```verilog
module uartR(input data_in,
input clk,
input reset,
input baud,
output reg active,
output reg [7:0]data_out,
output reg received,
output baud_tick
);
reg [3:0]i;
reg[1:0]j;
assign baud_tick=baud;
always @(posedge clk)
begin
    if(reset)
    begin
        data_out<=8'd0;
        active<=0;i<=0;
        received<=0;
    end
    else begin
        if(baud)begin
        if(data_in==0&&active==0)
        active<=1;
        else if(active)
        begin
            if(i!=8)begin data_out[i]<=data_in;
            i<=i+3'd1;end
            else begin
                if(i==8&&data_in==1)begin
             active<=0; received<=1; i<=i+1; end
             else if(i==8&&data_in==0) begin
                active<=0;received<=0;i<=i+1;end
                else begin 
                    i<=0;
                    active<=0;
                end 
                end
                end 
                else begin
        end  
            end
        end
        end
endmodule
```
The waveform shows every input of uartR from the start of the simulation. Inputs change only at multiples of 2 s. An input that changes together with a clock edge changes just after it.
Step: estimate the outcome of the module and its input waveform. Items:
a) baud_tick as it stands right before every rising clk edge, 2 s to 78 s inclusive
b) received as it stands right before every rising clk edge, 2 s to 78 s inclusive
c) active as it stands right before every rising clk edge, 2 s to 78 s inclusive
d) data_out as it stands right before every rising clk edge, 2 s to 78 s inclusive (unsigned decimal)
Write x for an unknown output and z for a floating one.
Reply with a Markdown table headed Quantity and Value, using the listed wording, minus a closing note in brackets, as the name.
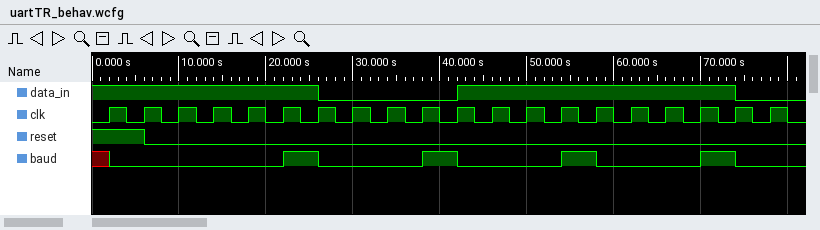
| Quantity | Value |
|---|---|
| baud_tick as it stands right before every rising clk edge, 2 s to 78 s inclusive | x 0 0 0 0 0 1 0 0 0 1 0 0 0 1 0 0 0 1 0 |
| received as it stands right before every rising clk edge, 2 s to 78 s inclusive | x 0 0 0 0 0 0 0 0 0 0 0 0 0 0 0 0 0 0 0 |
| active as it stands right before every rising clk edge, 2 s to 78 s inclusive | x 0 0 0 0 0 0 0 0 0 0 1 1 1 1 1 1 1 1 1 |
| data_out as it stands right before every rising clk edge, 2 s to 78 s inclusive | x, 0, 0, 0, 0, 0, 0, 0, 0, 0, 0, 0, 0, 0, 0, 1, 1, 1, 1, 3 |
